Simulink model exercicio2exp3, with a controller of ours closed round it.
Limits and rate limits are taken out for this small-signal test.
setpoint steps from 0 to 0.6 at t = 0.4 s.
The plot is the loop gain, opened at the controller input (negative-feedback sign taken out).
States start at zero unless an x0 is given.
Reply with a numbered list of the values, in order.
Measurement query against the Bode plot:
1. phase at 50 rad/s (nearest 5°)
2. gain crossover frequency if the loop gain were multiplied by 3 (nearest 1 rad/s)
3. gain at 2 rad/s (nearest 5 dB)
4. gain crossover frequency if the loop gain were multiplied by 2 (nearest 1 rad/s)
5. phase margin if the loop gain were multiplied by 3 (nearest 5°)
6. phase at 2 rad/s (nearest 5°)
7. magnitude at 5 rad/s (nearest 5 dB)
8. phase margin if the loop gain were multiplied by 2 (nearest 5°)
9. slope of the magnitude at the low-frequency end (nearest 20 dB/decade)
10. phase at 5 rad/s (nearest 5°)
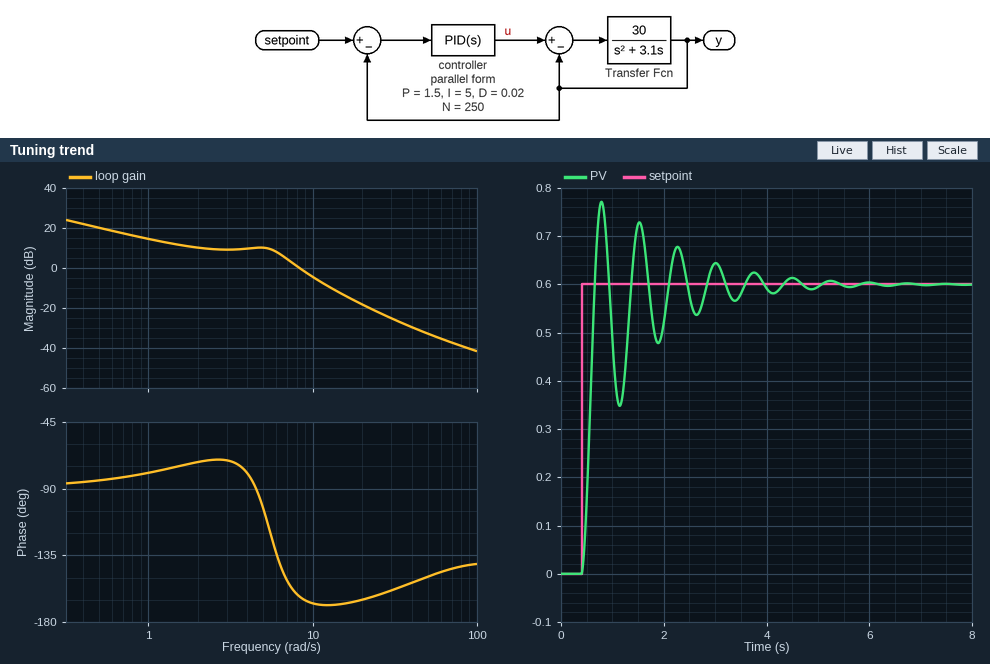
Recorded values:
1. -150°
2. 13 rad/s
3. 10 dB
4. 11 rad/s
5. 10°
6. -70°
7. 10 dB
8. 10°
9. -20 dB/decade
10. -105°
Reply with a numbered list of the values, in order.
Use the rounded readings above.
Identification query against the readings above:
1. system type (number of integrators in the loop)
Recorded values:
1. 1
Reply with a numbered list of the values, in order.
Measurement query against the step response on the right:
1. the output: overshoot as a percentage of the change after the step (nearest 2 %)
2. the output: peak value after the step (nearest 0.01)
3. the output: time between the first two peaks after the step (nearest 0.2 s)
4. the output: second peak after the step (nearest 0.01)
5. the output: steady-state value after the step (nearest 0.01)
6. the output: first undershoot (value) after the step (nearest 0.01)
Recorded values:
1. 28 %
2. 0.77
3. 0.8 s
4. 0.73
5. 0.60
6. 0.35
